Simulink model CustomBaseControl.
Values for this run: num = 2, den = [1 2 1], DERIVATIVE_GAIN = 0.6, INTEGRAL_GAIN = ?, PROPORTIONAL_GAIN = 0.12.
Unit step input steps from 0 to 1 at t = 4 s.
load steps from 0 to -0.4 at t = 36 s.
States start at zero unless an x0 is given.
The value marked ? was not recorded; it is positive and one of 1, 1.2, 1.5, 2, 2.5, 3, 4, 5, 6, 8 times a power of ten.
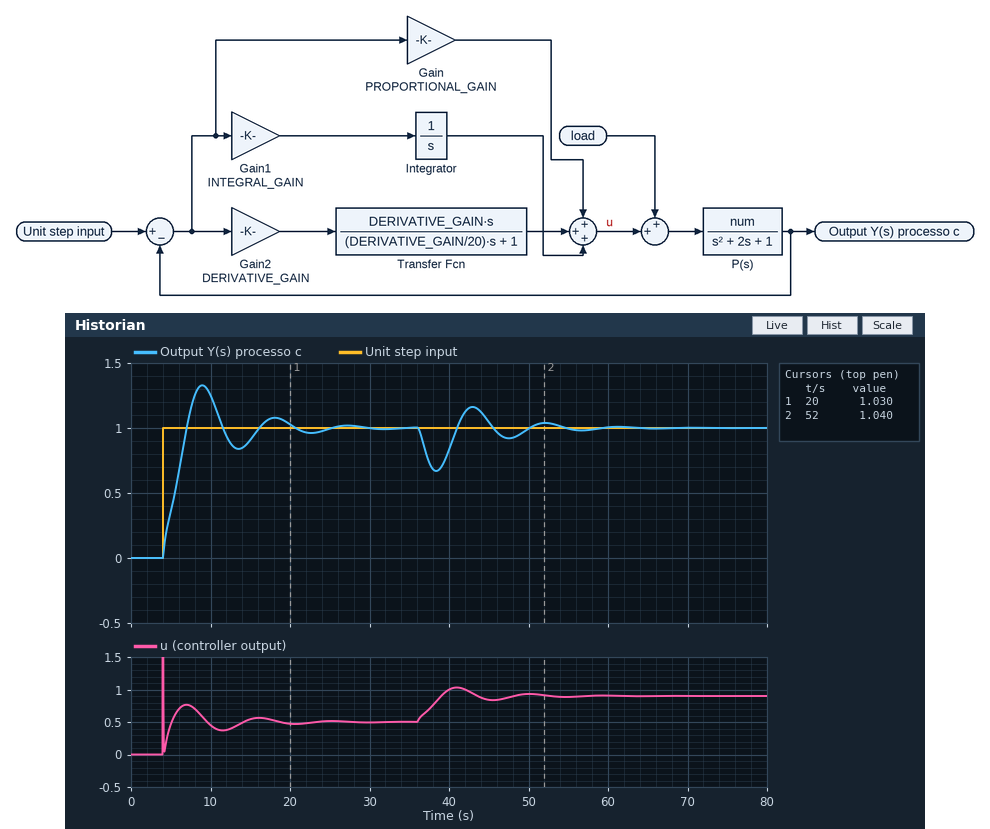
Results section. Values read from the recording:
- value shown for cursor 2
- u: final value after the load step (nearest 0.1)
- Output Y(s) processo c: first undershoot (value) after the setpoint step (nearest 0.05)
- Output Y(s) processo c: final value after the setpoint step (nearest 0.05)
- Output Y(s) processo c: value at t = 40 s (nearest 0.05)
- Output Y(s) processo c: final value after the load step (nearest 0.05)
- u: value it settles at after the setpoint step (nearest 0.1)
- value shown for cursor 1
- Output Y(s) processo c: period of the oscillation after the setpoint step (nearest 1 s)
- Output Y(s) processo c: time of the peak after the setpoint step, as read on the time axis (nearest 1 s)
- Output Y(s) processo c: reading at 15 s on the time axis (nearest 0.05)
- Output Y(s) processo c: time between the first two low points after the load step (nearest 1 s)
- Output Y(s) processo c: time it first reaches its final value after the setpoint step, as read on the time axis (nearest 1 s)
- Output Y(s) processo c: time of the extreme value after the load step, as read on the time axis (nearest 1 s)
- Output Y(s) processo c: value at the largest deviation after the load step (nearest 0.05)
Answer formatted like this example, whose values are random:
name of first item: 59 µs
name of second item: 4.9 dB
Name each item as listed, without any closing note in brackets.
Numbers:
value shown for cursor 2: 1.040
u: final value after the load step: 0.9
Output Y(s) processo c: first undershoot (value) after the setpoint step: 0.85
Output Y(s) processo c: final value after the setpoint step: 1.00
Output Y(s) processo c: value at t = 40 s: 0.85
Output Y(s) processo c: final value after the load step: 1.00
u: value it settles at after the setpoint step: 0.5
value shown for cursor 1: 1.030
Output Y(s) processo c: period of the oscillation after the setpoint step: 9 s
Output Y(s) processo c: time of the peak after the setpoint step, as read on the time axis: 9 s
Output Y(s) processo c: reading at 15 s on the time axis: 0.90
Output Y(s) processo c: time between the first two low points after the load step: 9 s
Output Y(s) processo c: time it first reaches its final value after the setpoint step, as read on the time axis: 7 s
Output Y(s) processo c: time of the extreme value after the load step, as read on the time axis: 38 s
Output Y(s) processo c: value at the largest deviation after the load step: 0.65
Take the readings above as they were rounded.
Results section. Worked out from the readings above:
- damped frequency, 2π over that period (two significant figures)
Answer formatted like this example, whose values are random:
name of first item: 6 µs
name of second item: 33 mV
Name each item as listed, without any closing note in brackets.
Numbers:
damped frequency, 2π over that period: 0.70 rad/s
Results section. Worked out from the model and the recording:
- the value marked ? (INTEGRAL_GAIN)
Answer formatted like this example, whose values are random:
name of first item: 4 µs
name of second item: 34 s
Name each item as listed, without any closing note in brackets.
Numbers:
the value marked ?: 0.6
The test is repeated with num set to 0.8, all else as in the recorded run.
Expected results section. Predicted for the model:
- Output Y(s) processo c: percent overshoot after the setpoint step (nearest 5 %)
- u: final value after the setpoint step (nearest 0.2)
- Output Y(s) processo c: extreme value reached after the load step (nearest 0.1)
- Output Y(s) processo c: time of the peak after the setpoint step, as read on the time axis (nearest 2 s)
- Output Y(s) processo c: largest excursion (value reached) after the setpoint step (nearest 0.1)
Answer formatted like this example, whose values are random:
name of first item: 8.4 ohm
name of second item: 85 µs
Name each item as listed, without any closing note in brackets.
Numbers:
Output Y(s) processo c: percent overshoot after the setpoint step: 15 %
u: final value after the setpoint step: 1.2
Output Y(s) processo c: extreme value reached after the load step: 0.8
Output Y(s) processo c: time of the peak after the setpoint step, as read on the time axis: 12 s
Output Y(s) processo c: largest excursion (value reached) after the setpoint step: 1.2
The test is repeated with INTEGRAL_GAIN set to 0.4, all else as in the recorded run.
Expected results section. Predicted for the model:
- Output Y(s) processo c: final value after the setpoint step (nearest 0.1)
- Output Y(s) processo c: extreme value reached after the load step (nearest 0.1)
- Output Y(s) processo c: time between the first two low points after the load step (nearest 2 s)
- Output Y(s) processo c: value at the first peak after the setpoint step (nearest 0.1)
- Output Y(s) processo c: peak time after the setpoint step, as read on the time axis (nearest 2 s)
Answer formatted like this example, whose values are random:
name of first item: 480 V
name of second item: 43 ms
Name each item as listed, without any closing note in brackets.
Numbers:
Output Y(s) processo c: final value after the setpoint step: 1.0
Output Y(s) processo c: extreme value reached after the load step: 0.6
Output Y(s) processo c: time between the first two low points after the load step: 12 s
Output Y(s) processo c: value at the first peak after the setpoint step: 1.2
Output Y(s) processo c: peak time after the setpoint step, as read on the time axis: 10 s
